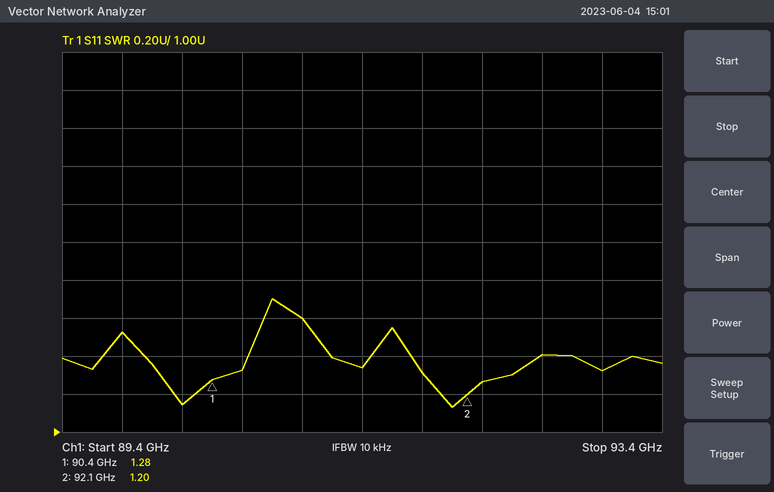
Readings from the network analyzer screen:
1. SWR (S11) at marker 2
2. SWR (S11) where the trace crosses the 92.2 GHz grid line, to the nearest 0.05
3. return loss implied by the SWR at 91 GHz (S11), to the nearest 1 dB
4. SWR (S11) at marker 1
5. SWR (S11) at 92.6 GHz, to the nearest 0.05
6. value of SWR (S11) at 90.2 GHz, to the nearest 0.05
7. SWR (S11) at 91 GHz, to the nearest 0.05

1.20
1.25
13 dB
1.28
1.40
1.15
1.60
